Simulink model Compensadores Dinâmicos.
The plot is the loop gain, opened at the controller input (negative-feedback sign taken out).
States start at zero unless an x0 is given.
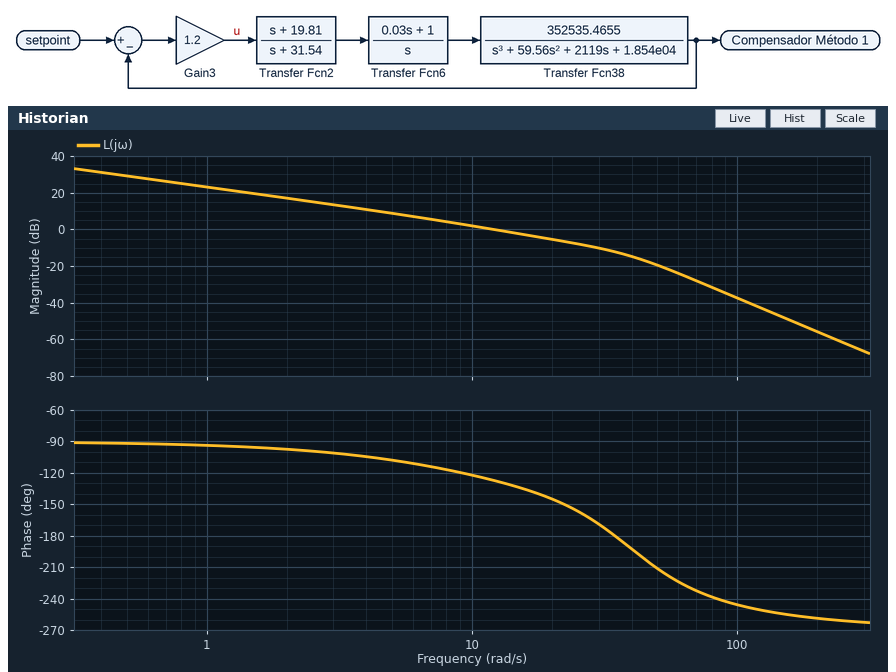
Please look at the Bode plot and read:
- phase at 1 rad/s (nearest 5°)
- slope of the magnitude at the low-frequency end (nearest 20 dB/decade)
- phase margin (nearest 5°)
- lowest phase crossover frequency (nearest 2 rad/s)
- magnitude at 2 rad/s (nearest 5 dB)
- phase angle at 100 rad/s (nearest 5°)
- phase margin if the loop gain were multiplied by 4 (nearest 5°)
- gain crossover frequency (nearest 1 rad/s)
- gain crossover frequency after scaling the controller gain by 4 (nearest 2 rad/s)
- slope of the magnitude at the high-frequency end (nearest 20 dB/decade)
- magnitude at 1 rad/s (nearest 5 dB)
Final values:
-95°
-20 dB/decade
55°
34 rad/s
15 dB
-245°
0°
12 rad/s
34 rad/s
-60 dB/decade
25 dB
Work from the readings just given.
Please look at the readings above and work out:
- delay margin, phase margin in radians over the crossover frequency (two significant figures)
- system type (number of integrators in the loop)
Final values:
0.080 s
1
